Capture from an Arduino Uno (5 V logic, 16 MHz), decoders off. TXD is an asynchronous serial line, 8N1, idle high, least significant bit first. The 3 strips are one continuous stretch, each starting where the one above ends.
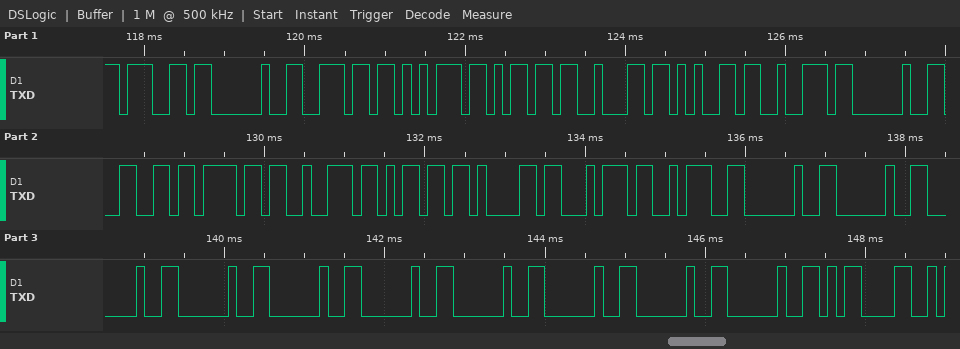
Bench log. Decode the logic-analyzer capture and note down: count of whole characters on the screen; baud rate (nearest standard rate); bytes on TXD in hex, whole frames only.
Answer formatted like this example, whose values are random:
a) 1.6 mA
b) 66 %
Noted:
a) 27
b) 9600 baud
c) 67 20 6E 75 6D 62 65 72 20 66 6F 72 6D 61 74 3A 20 20 20 20 20 20 20 20 20 20 0D
